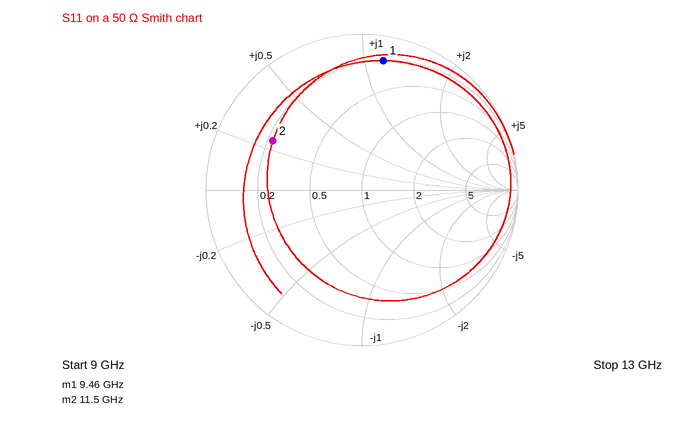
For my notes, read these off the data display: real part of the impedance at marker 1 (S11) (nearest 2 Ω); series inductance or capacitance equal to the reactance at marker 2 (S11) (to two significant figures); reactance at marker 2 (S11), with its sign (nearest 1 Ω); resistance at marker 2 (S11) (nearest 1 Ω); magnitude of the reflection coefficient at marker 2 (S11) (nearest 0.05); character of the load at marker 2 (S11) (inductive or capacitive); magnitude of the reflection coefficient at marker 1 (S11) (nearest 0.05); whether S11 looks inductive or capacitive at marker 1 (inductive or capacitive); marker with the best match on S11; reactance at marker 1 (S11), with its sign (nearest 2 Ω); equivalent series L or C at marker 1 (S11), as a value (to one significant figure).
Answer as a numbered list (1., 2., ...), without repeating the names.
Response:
1. 10 Ω
2. 170 pH
3. +12 Ω
4. 11 Ω
5. 0.65
6. inductive
7. 0.85
8. inductive
9. marker 2
10. +58 Ω
11. 1.0 nH
